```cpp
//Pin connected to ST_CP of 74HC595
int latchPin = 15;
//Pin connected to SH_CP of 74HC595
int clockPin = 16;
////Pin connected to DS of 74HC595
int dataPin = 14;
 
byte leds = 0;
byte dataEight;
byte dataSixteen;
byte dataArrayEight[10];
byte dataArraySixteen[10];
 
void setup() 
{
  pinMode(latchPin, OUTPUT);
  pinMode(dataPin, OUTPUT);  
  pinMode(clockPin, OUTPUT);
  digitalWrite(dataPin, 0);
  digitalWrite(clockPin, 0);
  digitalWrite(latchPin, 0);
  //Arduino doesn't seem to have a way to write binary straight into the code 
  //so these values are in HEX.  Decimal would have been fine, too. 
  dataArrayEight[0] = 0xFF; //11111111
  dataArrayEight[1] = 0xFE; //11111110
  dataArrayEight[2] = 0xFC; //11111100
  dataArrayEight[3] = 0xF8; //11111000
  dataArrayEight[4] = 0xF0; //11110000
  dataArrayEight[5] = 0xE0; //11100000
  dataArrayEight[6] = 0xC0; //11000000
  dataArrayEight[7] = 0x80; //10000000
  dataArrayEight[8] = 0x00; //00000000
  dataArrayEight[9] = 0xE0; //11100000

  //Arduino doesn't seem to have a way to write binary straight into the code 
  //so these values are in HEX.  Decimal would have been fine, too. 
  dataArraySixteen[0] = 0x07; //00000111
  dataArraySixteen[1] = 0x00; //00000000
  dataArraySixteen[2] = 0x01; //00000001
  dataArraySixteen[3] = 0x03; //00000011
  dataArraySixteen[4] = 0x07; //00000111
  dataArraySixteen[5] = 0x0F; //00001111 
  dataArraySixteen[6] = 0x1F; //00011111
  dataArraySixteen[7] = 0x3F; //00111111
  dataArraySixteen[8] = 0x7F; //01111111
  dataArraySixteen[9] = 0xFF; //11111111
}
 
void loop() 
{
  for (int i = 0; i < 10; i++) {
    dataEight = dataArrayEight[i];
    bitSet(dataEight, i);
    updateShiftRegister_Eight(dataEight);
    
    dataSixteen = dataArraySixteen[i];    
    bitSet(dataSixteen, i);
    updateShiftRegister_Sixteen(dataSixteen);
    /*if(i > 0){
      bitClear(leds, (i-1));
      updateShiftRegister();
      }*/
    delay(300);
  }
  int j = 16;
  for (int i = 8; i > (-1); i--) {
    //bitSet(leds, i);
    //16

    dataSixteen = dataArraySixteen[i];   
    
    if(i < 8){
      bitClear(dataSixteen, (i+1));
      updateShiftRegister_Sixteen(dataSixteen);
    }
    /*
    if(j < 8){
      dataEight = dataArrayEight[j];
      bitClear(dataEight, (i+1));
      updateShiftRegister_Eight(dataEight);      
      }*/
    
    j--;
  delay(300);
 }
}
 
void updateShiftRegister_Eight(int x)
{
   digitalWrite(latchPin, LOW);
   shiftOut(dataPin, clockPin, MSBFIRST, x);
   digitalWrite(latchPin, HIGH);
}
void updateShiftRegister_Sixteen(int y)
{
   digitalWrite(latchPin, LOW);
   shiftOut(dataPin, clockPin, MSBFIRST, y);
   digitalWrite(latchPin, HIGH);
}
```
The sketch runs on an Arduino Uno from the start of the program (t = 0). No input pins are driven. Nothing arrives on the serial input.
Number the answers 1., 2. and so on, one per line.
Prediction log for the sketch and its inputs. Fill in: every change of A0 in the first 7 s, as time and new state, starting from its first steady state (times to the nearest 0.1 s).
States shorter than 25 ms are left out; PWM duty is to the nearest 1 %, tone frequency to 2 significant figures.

1. 0 s high; 0.3 s low; 0.6 s high; 5.1 s low; 5.4 s high; 6 s low; 6.3 s high
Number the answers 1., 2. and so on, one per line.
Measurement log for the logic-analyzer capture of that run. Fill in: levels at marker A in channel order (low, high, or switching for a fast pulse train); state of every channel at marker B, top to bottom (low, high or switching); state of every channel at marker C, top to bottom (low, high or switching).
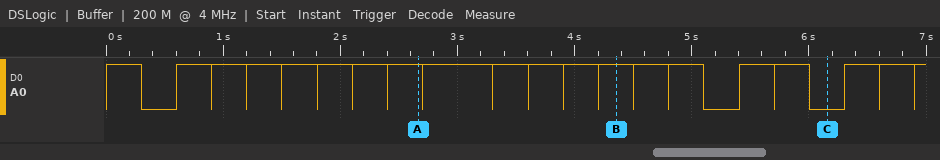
1. A0 high
2. A0 high
3. A0 low
